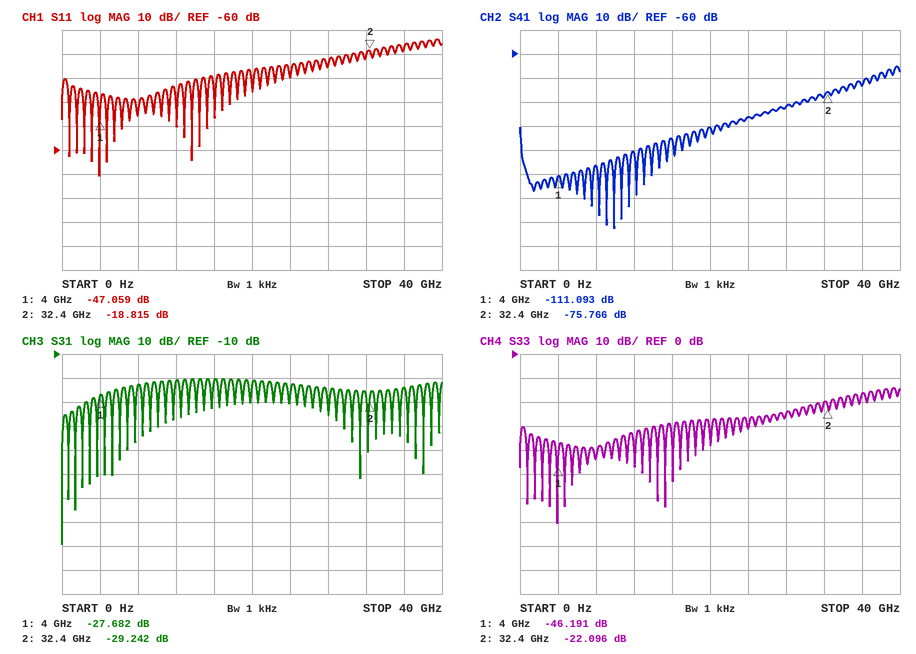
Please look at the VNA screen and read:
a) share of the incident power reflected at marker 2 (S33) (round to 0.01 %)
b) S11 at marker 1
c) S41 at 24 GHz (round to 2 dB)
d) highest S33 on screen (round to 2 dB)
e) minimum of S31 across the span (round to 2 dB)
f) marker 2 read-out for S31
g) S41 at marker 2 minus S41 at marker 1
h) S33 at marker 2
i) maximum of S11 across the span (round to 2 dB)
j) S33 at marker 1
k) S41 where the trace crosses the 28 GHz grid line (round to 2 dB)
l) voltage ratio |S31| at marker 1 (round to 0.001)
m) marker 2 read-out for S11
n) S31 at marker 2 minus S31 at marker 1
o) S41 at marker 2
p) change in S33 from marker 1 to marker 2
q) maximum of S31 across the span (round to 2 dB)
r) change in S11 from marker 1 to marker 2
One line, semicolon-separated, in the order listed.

0.62 %; -47.059 dB; -86 dB; -14 dB; -90 dB; -29.242 dB; 35.327 dB; -22.096 dB; -14 dB; -46.191 dB; -82 dB; 0.041; -18.815 dB; -1.560 dB; -75.766 dB; 24.095 dB; -20 dB; 28.244 dB
